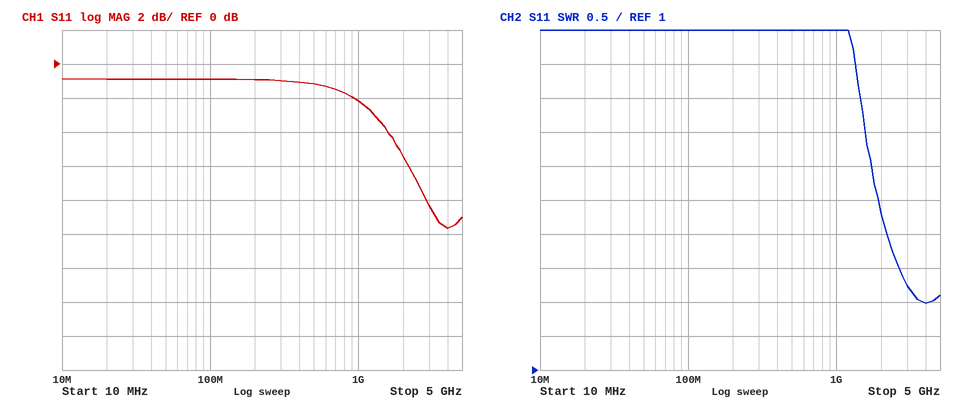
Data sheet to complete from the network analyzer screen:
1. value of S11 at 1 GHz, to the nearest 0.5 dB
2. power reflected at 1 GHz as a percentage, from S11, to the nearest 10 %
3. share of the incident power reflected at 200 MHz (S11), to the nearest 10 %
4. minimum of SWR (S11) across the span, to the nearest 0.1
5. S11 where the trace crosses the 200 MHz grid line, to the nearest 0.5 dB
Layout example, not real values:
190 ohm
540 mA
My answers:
-2.0 dB
60 %
80 %
2.0
-1.0 dB
